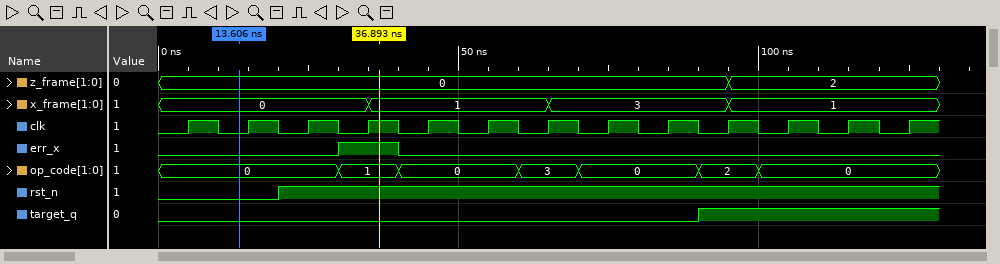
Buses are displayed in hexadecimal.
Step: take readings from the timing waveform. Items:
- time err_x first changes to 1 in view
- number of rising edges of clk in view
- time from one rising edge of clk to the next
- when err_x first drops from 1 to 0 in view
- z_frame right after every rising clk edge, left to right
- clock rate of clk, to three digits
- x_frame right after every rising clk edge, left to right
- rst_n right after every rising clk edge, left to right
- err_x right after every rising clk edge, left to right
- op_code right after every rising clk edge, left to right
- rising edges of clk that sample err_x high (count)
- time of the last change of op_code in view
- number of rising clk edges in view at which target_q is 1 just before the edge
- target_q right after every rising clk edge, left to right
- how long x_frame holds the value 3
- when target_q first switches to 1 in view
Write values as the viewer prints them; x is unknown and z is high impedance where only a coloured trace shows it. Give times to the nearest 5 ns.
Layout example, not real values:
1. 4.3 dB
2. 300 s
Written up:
1. 30 ns
2. 13
3. 10 ns
4. 40 ns
5. 0, 0, 0, 0, 0, 0, 0, 0, 0, 2, 2, 2, 2
6. 100 MHz
7. 0, 0, 0, 1, 1, 1, 3, 3, 3, 1, 1, 1, 1
8. 0 0 1 1 1 1 1 1 1 1 1 1 1
9. 0 0 0 1 0 0 0 0 0 0 0 0 0
10. 0, 0, 0, 1, 0, 0, 3, 0, 0, 2, 0, 0, 0
11. 1
12. 100 ns
13. 4
14. 0 0 0 0 0 0 0 0 0 1 1 1 1
15. 30 ns
16. 90 ns
